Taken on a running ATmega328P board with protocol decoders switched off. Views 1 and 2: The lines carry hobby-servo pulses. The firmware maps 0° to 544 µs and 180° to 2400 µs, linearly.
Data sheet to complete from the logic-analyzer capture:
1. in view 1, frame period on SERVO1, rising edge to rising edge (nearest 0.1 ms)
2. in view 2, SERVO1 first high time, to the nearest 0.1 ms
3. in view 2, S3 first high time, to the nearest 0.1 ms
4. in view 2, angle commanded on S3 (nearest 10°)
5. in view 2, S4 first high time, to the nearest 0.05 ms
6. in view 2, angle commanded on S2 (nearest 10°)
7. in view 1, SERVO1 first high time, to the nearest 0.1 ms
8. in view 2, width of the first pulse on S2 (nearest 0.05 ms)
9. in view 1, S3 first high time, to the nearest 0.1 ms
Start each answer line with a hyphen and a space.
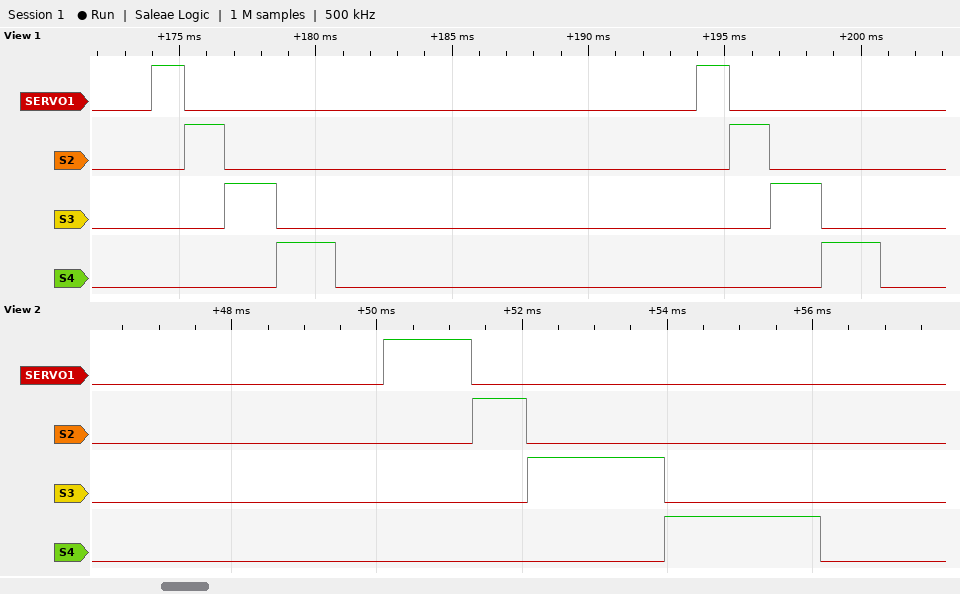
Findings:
- 20.0 ms
- 1.2 ms
- 1.9 ms
- 130°
- 2.15 ms
- 20°
- 1.2 ms
- 0.75 ms
- 1.9 ms
